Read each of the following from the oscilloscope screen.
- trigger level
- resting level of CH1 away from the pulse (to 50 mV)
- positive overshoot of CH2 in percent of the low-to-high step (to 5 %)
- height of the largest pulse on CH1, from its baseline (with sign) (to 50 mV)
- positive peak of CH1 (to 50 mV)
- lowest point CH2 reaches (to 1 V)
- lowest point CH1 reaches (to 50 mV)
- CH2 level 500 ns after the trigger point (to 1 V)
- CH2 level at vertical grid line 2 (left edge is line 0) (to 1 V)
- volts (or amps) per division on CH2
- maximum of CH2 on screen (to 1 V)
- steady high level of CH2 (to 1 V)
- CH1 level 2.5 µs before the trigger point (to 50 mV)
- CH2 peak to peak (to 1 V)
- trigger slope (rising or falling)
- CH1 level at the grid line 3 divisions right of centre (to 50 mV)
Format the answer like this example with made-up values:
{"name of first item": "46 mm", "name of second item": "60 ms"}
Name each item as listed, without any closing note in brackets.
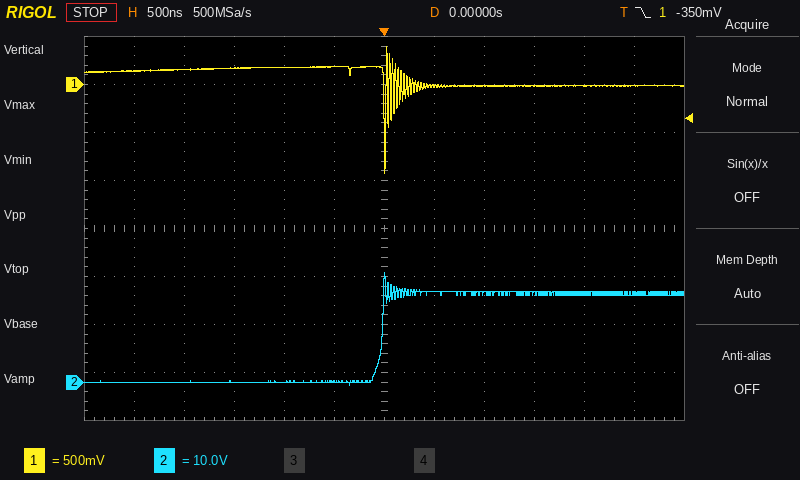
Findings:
{"trigger level": "-350 mV", "resting level of CH1 away from the pulse": "150 mV", "positive overshoot of CH2 in percent of the low-to-high step": "20 %", "height of the largest pulse on CH1, from its baseline (with sign)": "-1.10 V", "positive peak of CH1": "400 mV", "lowest point CH2 reaches": "-1 V", "lowest point CH1 reaches": "-950 mV", "CH2 level 500 ns after the trigger point": "19 V", "CH2 level at vertical grid line 2 (left edge is line 0)": "0 V", "volts (or amps) per division on CH2": "10 V", "maximum of CH2 on screen": "23 V", "steady high level of CH2": "19 V", "CH1 level 2.5 µs before the trigger point": "150 mV", "CH2 peak to peak": "24 V", "trigger slope": "falling", "CH1 level at the grid line 3 divisions right of centre": "0 mV"}
